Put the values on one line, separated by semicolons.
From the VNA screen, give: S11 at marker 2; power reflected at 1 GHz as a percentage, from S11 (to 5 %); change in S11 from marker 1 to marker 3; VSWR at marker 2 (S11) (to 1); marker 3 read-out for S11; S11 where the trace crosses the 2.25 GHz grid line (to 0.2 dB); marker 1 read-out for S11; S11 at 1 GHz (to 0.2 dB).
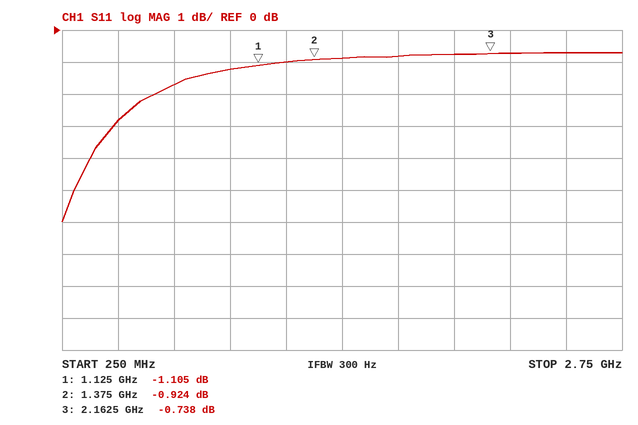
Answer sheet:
-0.924 dB; 75 %; 0.367 dB; 19; -0.738 dB; -0.8 dB; -1.105 dB; -1.2 dB
